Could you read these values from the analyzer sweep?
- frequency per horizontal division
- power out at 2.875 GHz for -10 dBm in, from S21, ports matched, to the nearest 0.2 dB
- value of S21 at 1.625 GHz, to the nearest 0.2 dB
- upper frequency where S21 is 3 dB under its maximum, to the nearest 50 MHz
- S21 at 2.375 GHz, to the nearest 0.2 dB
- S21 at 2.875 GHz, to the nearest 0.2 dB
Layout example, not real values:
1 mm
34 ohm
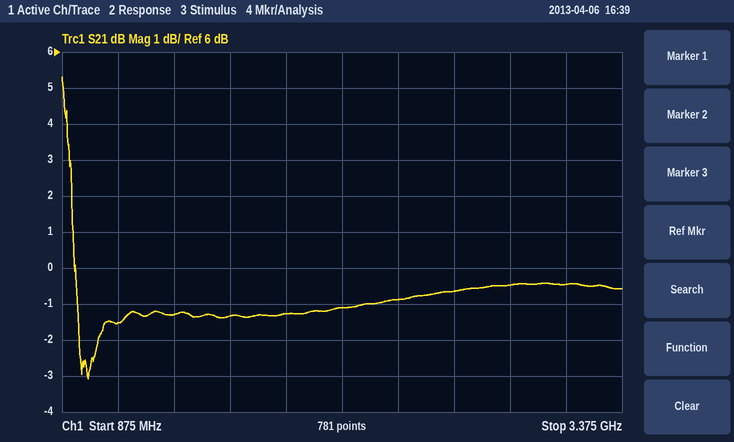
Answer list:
250 MHz
-10.4 dBm
-1.4 dB
900 MHz
-0.8 dB
-0.4 dB
